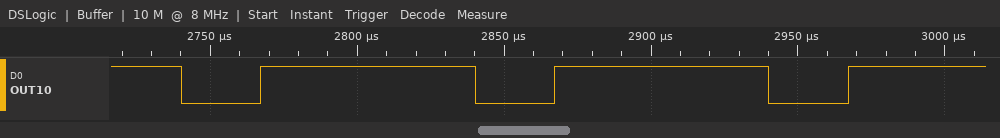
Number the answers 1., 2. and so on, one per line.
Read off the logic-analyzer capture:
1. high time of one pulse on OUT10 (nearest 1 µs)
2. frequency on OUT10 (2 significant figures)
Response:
1. 73 µs
2. 10 kHz
